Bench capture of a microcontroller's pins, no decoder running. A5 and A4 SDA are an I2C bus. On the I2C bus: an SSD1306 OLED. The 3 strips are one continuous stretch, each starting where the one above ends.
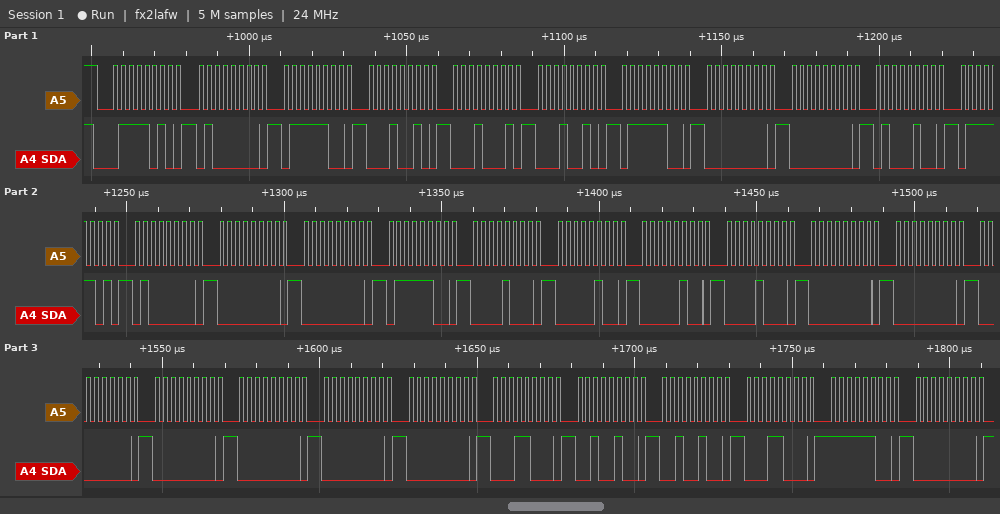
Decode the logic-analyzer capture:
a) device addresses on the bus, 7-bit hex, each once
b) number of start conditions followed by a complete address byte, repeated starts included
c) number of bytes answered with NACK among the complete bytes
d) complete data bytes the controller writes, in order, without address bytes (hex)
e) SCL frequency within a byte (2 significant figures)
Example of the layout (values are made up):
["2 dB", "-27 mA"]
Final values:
["0x3D", "1", "0", "40 7C 12 11 12 7C 00 00 44 7D 40 00 00 7C 08 04 04 08 00 00 00 00 00 00 00 18 24 24 18 FC 00", "400 kHz"]
